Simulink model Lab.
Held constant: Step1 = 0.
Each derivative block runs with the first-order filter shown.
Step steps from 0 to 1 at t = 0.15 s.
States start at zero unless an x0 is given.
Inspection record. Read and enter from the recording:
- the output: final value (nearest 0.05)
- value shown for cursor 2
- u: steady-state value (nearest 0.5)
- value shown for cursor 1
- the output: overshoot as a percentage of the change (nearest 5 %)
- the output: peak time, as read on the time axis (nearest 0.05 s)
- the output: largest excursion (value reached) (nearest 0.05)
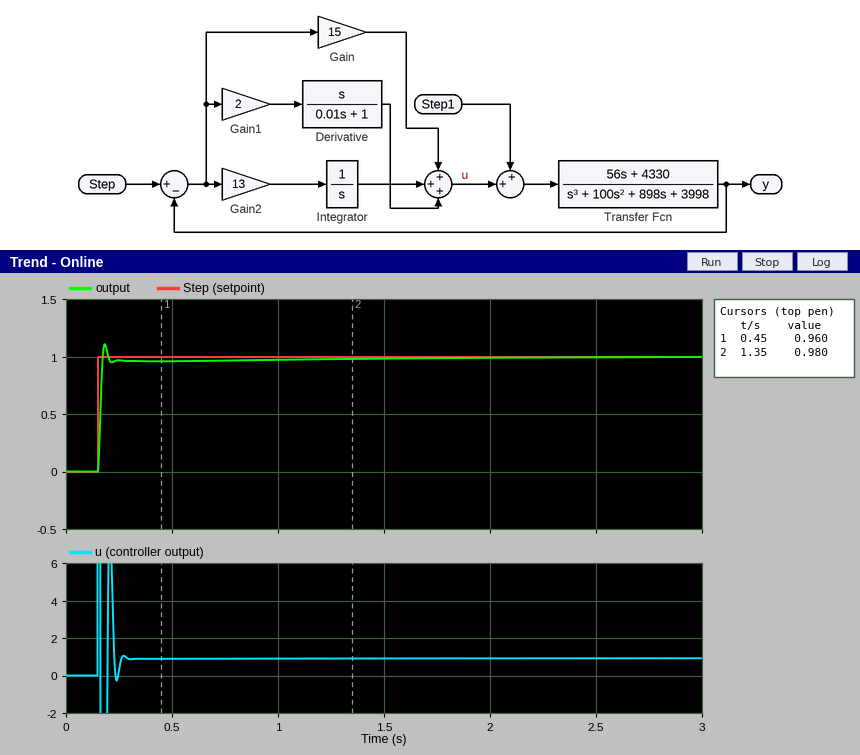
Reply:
1.00
0.980
1.0
0.960
10 %
0.20 s
1.10
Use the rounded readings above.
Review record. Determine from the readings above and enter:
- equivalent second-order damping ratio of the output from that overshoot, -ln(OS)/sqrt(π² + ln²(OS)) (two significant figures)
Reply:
0.59
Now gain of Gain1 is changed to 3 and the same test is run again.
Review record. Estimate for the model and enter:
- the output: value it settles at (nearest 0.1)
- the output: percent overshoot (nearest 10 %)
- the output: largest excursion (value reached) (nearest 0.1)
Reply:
1.0
20 %
1.2
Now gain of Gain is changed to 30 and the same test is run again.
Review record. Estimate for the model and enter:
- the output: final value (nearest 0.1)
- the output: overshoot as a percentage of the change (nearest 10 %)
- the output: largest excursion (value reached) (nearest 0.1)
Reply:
1.0
20 %
1.2
